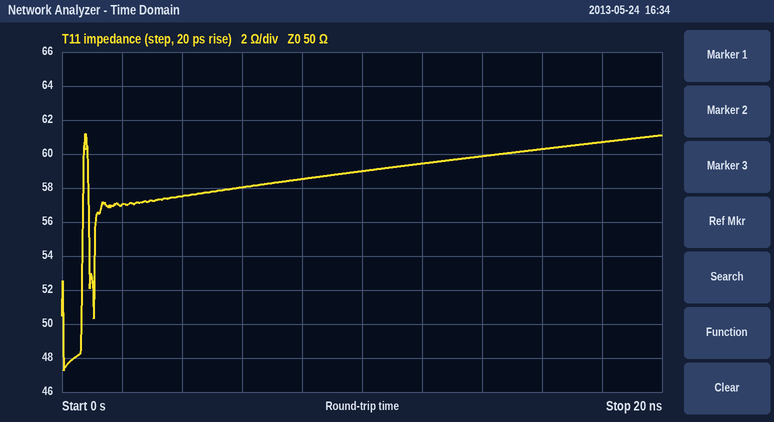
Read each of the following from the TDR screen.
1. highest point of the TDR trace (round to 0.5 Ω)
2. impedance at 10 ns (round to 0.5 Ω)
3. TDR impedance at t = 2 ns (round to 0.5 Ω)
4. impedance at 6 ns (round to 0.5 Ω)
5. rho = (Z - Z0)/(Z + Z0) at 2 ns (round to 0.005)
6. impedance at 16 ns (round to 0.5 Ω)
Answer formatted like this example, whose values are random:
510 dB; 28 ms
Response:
61.0 Ω; 59.0 Ω; 57.0 Ω; 58.0 Ω; +0.065; 60.5 Ω
